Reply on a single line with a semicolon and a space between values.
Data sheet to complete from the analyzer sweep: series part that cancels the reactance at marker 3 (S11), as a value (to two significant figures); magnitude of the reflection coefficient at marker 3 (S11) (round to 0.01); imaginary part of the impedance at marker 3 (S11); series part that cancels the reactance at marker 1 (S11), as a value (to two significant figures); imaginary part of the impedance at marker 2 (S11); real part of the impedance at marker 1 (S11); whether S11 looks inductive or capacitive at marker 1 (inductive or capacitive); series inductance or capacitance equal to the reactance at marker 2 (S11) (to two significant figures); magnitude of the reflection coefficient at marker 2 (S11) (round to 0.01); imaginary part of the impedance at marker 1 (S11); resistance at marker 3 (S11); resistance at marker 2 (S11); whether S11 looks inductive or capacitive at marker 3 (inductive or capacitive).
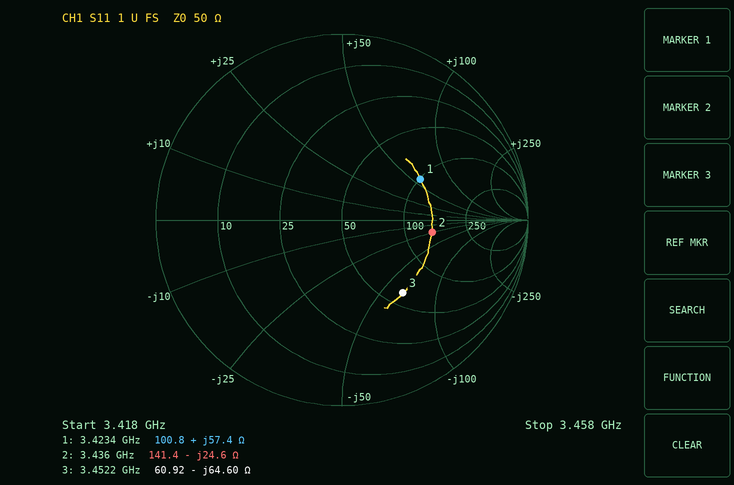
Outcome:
3.0 nH; 0.51; -64.60 Ω; 810 fF; -24.6 Ω; 100.8 Ω; inductive; 1.9 pF; 0.49; +57.4 Ω; 60.92 Ω; 141.4 Ω; capacitive
